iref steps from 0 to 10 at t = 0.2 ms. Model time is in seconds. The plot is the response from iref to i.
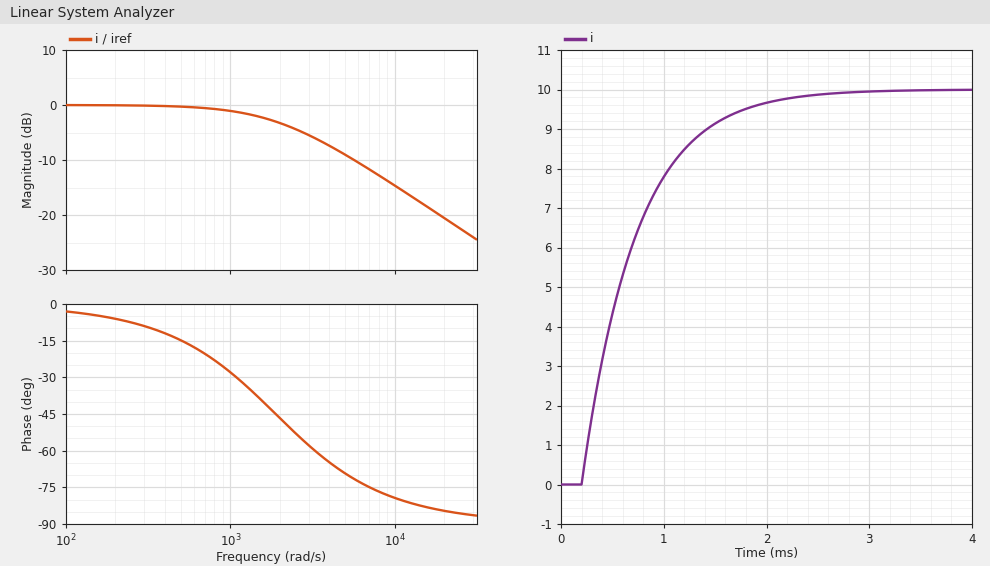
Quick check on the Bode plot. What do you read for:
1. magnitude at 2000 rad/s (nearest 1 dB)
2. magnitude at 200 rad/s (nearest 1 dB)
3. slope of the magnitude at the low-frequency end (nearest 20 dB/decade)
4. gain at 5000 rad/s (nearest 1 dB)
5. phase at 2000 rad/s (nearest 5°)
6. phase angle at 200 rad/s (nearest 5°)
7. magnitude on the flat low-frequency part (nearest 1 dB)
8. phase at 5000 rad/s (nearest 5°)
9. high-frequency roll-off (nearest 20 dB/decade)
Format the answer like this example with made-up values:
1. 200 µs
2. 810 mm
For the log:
1. -3 dB
2. 0 dB
3. 0 dB/decade
4. -9 dB
5. -45°
6. -5°
7. 0 dB
8. -70°
9. -20 dB/decade
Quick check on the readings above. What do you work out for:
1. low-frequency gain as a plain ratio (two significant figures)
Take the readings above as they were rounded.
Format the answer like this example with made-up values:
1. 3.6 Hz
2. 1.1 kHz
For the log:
1. 1.0
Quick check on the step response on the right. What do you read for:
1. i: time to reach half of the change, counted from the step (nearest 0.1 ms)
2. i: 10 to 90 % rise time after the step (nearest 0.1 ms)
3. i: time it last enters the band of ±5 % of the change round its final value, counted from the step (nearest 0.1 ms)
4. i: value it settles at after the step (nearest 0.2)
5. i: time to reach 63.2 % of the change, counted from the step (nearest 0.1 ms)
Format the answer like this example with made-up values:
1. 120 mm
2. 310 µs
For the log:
1. 0.4 ms
2. 1.2 ms
3. 1.6 ms
4. 10.0
5. 0.5 ms
